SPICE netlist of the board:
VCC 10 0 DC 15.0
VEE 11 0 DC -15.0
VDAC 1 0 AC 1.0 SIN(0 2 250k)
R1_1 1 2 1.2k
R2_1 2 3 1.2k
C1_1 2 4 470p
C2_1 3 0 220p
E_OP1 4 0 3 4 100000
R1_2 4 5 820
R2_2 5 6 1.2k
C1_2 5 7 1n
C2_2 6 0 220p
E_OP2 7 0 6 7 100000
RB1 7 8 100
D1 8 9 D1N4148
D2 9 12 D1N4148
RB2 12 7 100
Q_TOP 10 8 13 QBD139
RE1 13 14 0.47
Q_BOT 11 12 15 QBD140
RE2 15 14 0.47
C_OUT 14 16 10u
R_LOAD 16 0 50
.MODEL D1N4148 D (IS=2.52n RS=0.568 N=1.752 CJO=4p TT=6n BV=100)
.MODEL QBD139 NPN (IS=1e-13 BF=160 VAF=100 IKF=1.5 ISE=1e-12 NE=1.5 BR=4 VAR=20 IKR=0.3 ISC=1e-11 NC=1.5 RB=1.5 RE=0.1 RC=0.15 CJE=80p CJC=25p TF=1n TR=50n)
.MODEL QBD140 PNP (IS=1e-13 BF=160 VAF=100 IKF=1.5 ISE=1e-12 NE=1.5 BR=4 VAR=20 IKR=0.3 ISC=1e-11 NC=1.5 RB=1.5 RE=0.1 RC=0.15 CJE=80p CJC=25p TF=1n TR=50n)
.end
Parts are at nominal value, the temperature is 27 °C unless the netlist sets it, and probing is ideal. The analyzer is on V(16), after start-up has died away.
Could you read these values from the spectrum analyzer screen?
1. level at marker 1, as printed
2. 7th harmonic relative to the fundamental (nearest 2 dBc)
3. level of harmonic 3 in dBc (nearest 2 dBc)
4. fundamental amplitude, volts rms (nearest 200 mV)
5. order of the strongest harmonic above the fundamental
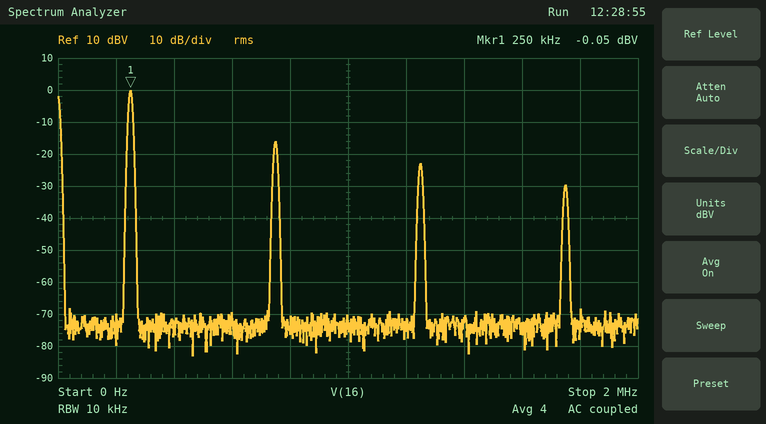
-0.05 dBV
-30 dBc
-16 dBc
1.0 V
3
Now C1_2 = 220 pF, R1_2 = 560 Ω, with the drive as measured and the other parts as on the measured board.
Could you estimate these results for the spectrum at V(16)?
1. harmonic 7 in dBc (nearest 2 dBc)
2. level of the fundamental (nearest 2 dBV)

-32 dBc
-4 dBV
